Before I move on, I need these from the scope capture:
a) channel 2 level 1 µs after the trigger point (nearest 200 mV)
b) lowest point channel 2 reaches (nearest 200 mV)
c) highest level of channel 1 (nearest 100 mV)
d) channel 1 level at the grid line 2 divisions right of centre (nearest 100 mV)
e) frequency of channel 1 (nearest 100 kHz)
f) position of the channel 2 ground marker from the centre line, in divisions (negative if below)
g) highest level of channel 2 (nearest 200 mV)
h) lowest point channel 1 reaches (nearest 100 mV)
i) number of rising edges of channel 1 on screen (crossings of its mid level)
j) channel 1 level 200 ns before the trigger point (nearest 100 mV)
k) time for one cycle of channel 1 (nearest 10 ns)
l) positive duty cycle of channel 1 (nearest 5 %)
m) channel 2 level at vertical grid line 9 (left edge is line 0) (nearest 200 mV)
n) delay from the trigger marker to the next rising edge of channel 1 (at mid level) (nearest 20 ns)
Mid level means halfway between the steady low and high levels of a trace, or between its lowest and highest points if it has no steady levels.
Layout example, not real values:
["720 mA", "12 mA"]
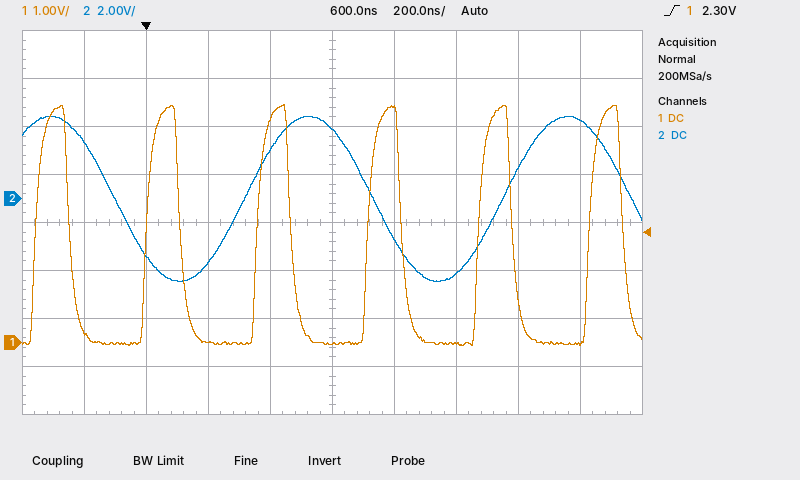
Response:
["-3.2 V", "-3.4 V", "5.0 V", "0.0 V", "2.8 MHz", "+0.5 div", "3.4 V", "-100 mV", "6", "200 mV", "360 ns", "30 %", "3.2 V", "360 ns"]
